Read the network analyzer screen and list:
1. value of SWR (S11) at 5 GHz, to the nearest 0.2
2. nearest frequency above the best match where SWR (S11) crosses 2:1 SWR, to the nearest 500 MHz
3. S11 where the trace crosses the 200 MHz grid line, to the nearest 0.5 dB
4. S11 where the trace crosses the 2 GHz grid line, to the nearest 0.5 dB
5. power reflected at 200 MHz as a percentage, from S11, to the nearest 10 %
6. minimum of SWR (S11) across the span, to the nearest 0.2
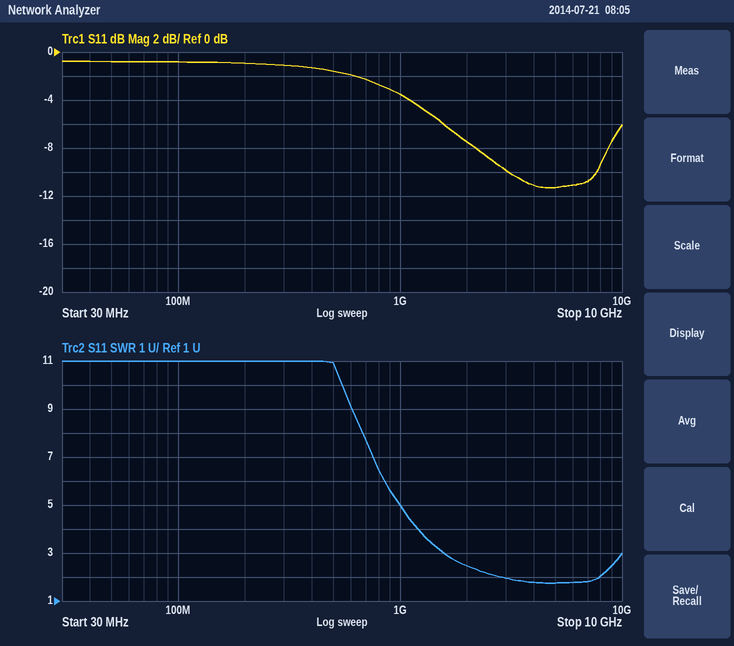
1.8
8.0 GHz
-1.0 dB
-7.5 dB
80 %
1.8
